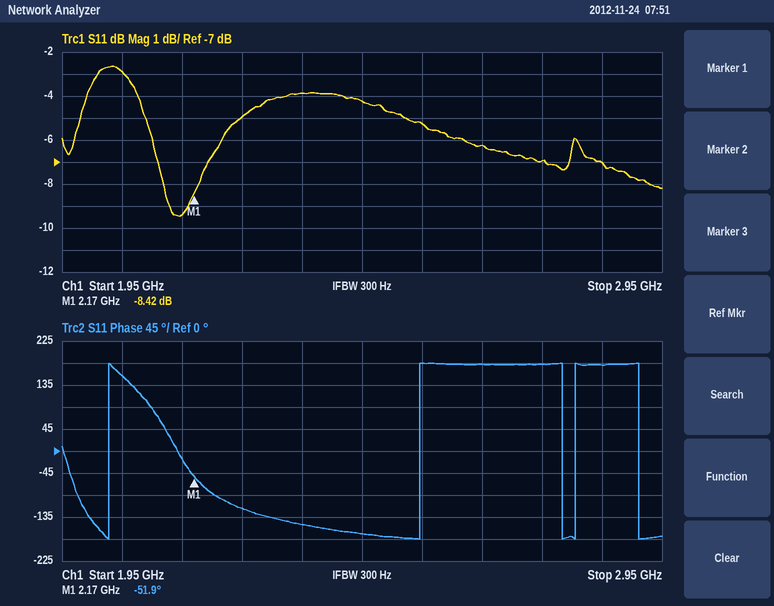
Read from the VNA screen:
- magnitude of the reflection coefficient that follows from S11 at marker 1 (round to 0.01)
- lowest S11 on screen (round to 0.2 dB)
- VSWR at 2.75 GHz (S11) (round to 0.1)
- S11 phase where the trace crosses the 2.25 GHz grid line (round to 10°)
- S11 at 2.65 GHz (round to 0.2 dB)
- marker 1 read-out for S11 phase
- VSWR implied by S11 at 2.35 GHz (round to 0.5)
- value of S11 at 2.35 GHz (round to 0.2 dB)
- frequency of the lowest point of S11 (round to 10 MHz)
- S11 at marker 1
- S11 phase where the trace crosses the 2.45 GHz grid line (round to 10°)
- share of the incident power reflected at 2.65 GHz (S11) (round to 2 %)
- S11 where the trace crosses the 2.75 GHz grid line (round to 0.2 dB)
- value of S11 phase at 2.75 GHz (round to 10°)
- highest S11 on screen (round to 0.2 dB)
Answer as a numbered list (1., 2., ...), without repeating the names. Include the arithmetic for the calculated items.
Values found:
1. 10^(-8.42/20) ≈ 0.38
2. -9.4 dB
3. |Γ| = 10^(-7/20) = 0.4467; VSWR = (1 + 0.4467)/(1 − 0.4467) ≈ 2.6
4. -120°
5. -6.2 dB
6. -51.9°
7. |Γ| = 10^(-3.8/20) = 0.6457; VSWR = (1 + 0.6457)/(1 − 0.6457) ≈ 4.64, so 4.5 to the nearest 0.5
8. -3.8 dB
9. 2.15 GHz
10. -8.42 dB
11. -170°
12. 10^(-6.2/10) ≈ 24 %
13. -7.0 dB
14. 180°
15. -2.6 dB
